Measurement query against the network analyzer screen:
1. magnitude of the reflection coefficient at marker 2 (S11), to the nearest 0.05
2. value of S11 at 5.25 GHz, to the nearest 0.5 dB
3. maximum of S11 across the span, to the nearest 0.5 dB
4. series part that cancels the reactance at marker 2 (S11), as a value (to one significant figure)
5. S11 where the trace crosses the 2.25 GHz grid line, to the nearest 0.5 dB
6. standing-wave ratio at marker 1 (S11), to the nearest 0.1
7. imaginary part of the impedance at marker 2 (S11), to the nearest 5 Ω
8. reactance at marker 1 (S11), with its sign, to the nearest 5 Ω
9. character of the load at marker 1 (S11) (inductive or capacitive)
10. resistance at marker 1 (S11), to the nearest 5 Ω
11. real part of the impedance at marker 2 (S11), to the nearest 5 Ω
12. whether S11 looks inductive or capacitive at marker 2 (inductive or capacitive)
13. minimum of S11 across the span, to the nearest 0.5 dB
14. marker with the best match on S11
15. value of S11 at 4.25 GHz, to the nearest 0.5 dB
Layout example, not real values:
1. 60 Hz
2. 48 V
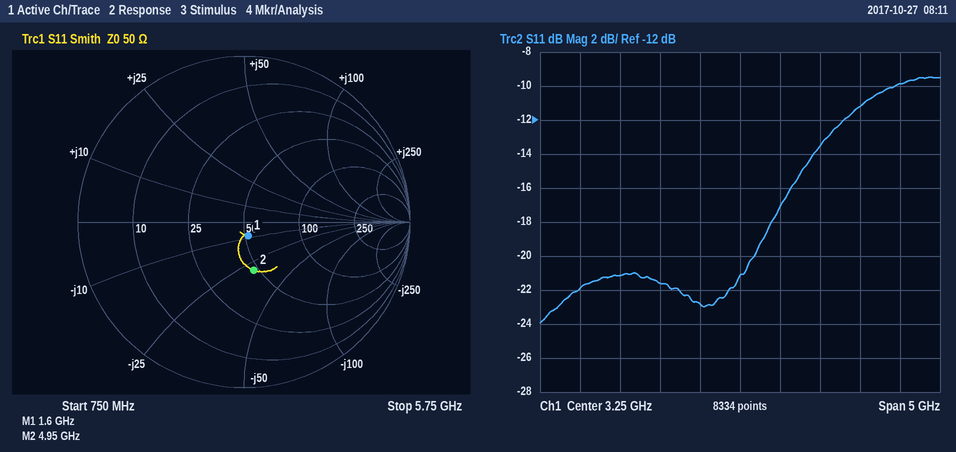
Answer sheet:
1. 0.30
2. -10.0 dB
3. -9.5 dB
4. 1.0 nH
5. -21.5 dB
6. 1.2
7. -30 Ω
8. -10 Ω
9. capacitive
10. 50 Ω
11. 45 Ω
12. capacitive
13. -24.0 dB
14. marker 1
15. -13.5 dB
